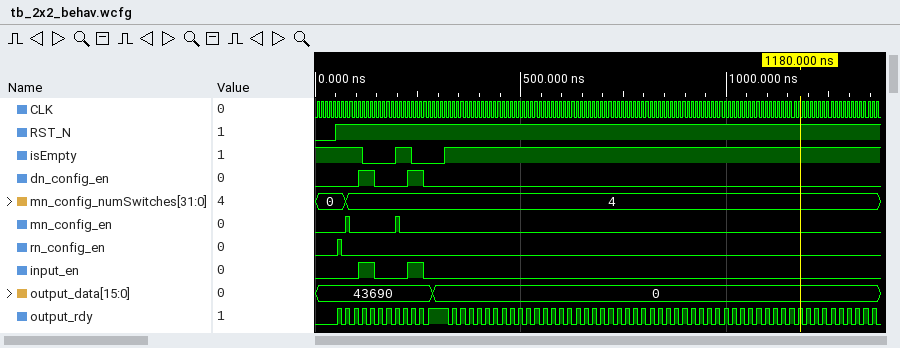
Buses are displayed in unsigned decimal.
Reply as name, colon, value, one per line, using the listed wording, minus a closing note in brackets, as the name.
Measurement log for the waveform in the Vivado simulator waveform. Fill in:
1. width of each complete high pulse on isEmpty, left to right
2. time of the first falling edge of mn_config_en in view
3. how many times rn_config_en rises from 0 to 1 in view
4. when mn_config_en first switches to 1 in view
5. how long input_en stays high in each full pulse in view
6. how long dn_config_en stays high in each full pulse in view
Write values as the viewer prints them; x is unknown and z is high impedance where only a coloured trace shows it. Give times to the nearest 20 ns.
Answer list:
width of each complete high pulse on isEmpty, left to right: 40 ns
time of the first falling edge of mn_config_en in view: 80 ns
how many times rn_config_en rises from 0 to 1 in view: 1
when mn_config_en first switches to 1 in view: 80 ns
how long input_en stays high in each full pulse in view: 40 ns, 40 ns
how long dn_config_en stays high in each full pulse in view: 40 ns, 40 ns
